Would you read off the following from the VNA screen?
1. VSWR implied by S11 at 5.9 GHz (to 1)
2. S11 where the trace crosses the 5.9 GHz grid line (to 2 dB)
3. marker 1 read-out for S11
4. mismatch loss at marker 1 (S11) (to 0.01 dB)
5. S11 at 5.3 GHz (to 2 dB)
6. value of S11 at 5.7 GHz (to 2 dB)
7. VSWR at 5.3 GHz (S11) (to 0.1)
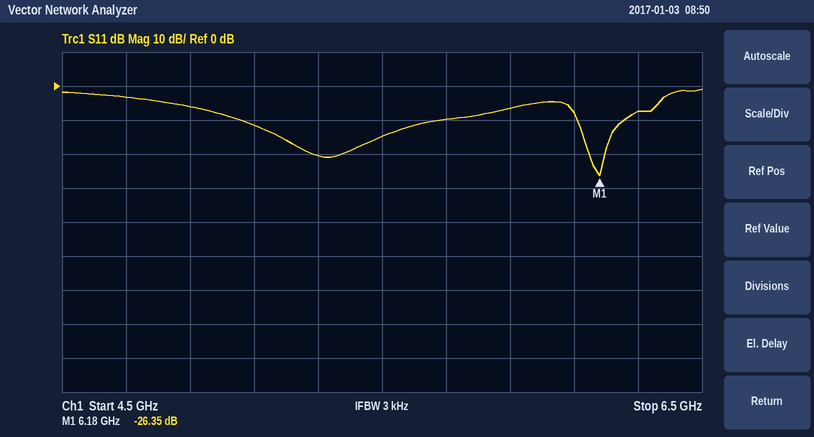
3
-6 dB
-26.35 dB
0.01 dB
-20 dB
-10 dB
1.2
